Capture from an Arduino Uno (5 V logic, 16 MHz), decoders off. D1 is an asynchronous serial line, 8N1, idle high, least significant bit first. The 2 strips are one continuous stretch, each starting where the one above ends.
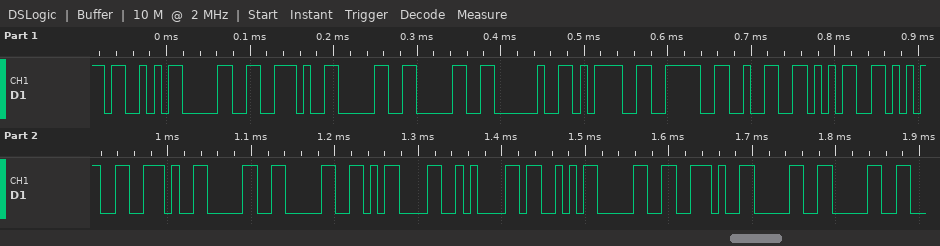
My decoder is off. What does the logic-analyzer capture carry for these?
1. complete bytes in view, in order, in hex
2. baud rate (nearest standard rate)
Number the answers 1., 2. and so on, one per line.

1. 53 30 2E 30 30 20 3D 3E 32 35 35 2E 30 30 0D 0A 53 30 2E 30 30
2. 115200 baud
